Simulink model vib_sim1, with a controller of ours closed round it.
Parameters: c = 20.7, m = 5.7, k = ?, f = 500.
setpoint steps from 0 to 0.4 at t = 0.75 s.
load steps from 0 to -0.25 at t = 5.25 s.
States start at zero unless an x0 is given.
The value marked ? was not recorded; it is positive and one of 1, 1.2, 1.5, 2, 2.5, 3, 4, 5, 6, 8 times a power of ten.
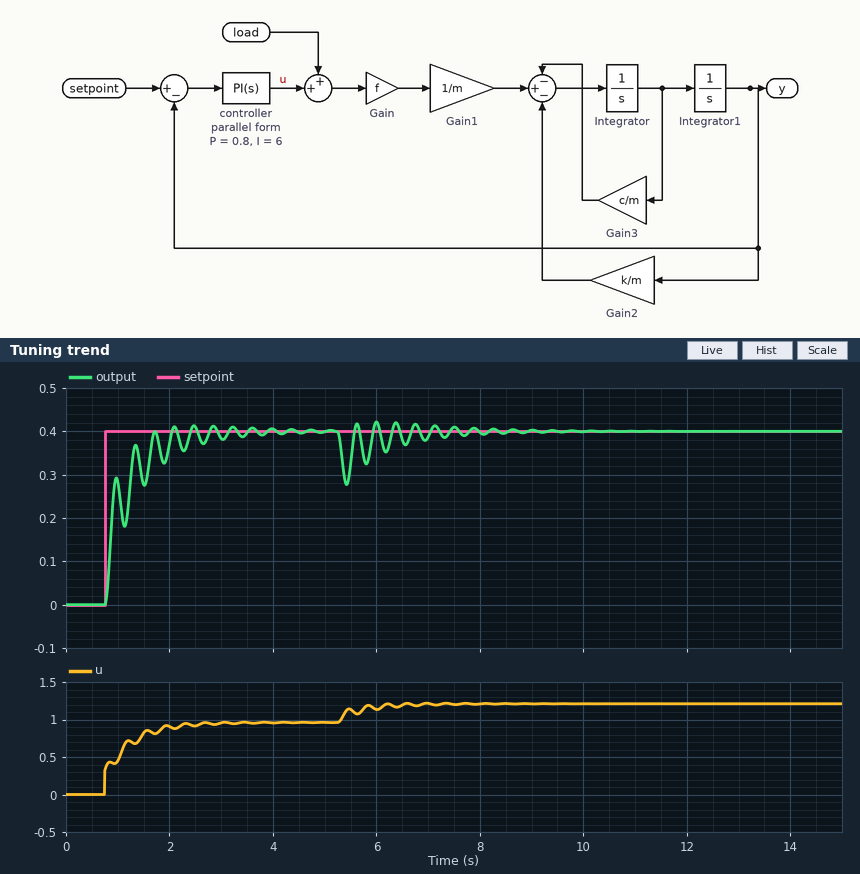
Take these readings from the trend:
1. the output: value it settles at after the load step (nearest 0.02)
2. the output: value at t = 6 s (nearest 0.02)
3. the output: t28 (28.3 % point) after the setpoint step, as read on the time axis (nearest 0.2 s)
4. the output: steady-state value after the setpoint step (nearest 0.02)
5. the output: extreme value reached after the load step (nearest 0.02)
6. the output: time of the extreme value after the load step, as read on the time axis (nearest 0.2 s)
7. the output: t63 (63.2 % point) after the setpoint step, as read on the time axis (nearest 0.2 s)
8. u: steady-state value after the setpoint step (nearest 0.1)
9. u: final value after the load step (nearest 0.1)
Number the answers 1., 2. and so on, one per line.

1. 0.40
2. 0.42
3. 0.8 s
4. 0.40
5. 0.28
6. 5.4 s
7. 1.0 s
8. 1.0
9. 1.2
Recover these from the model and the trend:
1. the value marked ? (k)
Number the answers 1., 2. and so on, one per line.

1. 1200
